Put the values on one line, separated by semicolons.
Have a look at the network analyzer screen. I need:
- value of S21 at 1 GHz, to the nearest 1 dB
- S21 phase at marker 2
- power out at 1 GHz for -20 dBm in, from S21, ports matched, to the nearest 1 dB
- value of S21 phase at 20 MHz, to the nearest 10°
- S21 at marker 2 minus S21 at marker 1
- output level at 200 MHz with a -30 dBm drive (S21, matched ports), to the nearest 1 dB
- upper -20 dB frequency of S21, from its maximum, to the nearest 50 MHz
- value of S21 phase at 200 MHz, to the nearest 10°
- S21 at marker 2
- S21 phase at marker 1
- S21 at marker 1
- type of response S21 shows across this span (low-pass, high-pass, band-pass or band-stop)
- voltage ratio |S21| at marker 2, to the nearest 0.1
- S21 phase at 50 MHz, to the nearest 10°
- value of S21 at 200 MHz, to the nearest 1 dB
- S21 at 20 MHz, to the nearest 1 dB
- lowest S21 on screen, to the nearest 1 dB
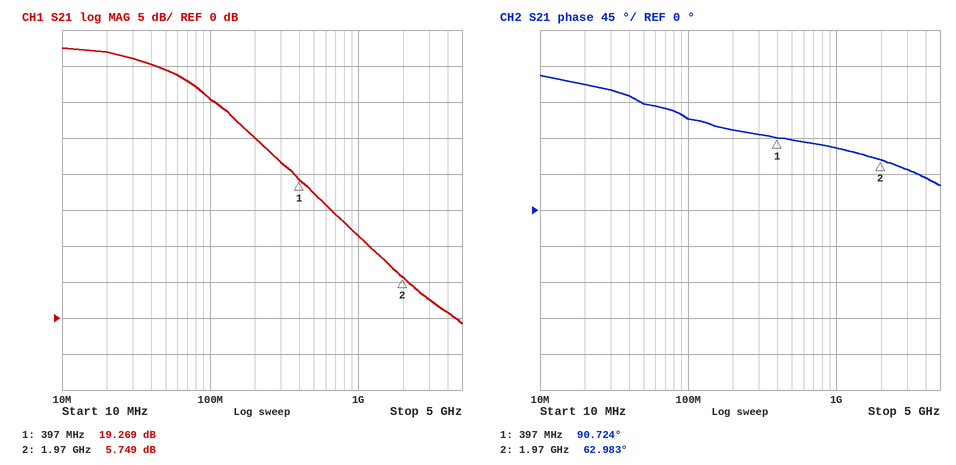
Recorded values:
11 dB; 62.983°; -9 dBm; 160°; -13.520 dB; -5 dBm; 500 MHz; 100°; 5.749 dB; 90.724°; 19.269 dB; low-pass; 1.9; 130°; 25 dB; 37 dB; -1 dB
